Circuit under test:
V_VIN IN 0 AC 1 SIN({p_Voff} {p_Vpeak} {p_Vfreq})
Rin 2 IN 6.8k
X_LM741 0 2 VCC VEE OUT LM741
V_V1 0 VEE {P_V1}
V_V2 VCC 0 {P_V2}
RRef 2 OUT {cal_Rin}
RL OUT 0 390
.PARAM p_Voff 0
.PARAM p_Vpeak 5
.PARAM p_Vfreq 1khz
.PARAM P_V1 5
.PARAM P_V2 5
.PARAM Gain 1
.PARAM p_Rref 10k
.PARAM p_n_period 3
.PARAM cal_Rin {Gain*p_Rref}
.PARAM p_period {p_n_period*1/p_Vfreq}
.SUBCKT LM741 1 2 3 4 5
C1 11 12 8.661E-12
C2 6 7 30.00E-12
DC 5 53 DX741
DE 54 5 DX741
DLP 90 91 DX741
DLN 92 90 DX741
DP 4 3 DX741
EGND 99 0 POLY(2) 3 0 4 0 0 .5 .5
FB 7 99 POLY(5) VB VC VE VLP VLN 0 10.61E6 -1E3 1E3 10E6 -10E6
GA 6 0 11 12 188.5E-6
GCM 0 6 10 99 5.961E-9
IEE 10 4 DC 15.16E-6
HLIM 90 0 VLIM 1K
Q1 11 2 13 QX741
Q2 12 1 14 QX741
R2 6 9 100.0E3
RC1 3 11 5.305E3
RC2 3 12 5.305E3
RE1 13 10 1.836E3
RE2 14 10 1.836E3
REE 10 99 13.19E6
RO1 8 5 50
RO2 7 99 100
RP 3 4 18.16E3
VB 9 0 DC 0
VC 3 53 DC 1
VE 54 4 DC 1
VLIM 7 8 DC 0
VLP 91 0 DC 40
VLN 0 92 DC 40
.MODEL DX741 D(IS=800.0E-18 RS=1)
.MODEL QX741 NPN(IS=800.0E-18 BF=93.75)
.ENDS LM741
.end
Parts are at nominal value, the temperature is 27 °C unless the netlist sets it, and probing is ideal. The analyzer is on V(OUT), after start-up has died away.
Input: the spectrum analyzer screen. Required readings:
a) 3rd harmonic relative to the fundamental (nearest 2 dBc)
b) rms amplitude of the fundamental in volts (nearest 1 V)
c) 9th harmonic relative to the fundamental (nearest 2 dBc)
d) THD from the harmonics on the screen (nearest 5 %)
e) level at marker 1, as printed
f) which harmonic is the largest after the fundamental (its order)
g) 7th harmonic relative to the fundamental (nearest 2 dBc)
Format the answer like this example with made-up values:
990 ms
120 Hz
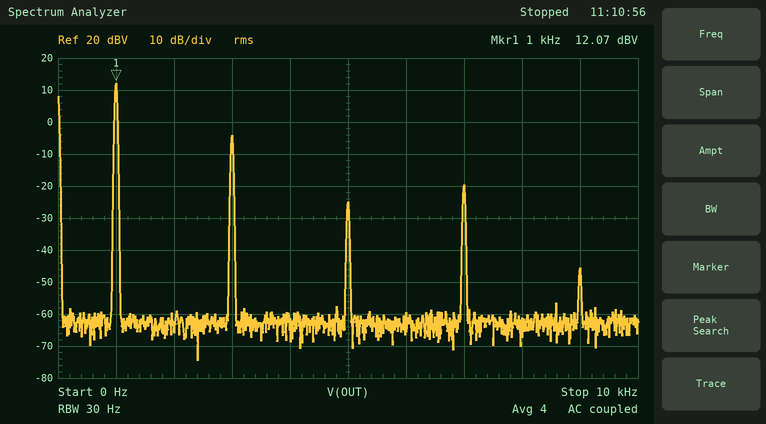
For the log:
-16 dBc
4 V
-58 dBc
15 %
12.07 dBV
3
-32 dBc
